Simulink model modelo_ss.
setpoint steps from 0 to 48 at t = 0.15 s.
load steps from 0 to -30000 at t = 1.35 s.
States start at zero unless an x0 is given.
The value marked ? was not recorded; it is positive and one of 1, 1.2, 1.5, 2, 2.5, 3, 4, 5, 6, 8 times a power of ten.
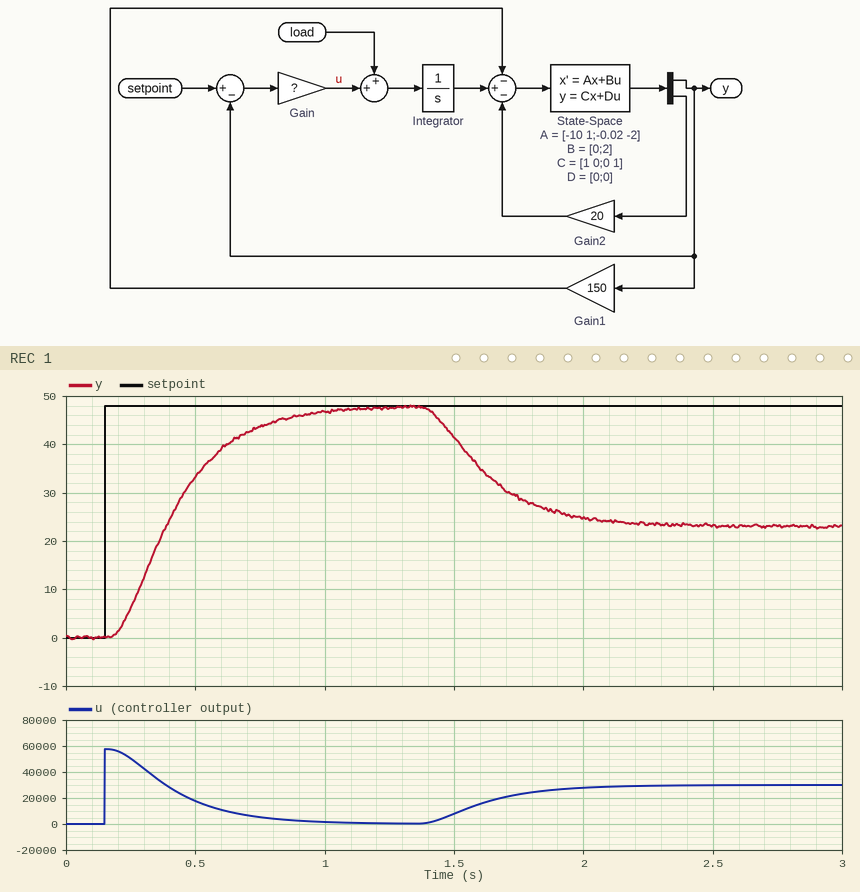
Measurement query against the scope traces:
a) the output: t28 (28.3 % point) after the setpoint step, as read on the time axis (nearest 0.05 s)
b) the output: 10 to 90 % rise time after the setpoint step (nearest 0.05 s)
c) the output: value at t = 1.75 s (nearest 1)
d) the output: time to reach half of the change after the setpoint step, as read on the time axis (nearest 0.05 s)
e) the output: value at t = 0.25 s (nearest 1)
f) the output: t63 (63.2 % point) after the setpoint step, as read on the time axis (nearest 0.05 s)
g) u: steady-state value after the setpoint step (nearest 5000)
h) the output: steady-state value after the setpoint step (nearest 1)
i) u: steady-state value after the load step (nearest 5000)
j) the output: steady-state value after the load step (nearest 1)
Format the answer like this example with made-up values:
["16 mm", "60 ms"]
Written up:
["0.30 s", "0.50 s", "29", "0.40 s", "6", "0.45 s", "0", "48", "30000", "23"]
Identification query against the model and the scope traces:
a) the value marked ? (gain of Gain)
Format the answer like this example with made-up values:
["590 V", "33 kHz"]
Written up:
["1200"]
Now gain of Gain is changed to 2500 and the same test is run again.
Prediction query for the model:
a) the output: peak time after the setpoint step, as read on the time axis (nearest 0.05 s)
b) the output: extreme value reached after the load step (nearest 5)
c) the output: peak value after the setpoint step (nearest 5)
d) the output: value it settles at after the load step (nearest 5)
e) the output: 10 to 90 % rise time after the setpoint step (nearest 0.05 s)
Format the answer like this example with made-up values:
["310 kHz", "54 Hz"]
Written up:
["0.55 s", "35", "50", "35", "0.20 s"]
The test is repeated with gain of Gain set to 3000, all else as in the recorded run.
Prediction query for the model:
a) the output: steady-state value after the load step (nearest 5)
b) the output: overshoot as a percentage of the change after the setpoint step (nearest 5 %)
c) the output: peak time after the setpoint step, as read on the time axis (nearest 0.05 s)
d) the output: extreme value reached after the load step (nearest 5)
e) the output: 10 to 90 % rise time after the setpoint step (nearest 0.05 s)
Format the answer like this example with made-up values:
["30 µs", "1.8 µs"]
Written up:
["40", "10 %", "0.50 s", "35", "0.15 s"]
